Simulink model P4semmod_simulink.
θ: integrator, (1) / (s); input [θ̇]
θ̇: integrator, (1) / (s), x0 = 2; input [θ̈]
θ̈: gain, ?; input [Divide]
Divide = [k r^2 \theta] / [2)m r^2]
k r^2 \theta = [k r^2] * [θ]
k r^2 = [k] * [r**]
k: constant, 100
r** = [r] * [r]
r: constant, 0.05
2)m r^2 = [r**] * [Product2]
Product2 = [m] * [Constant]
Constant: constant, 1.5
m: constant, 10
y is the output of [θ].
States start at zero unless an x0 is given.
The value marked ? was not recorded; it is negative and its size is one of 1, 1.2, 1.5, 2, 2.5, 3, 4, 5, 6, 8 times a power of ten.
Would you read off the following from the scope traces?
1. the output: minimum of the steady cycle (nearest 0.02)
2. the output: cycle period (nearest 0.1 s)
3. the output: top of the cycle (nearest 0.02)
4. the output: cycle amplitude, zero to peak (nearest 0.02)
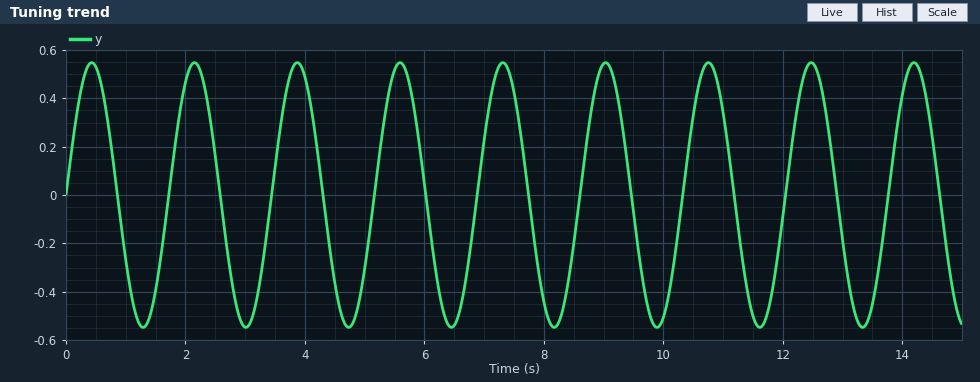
-0.54
1.7 s
0.54
0.54
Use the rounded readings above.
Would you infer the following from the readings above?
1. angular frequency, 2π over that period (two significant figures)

3.7 rad/s
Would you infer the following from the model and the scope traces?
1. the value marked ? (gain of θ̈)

-2
